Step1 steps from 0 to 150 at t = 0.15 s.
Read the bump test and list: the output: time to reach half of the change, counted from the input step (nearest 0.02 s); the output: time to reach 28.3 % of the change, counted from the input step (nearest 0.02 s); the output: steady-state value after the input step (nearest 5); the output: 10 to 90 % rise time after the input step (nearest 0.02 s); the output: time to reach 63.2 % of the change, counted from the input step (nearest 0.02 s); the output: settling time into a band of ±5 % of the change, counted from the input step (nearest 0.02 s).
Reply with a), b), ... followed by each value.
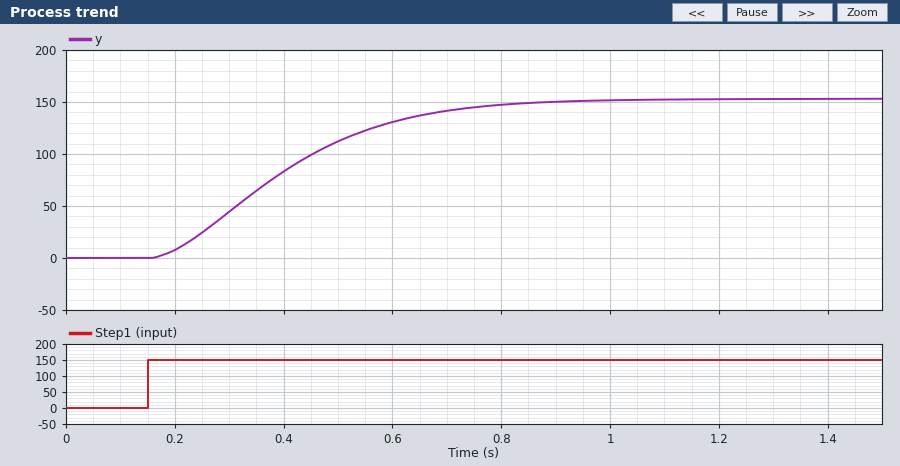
a) 0.24 s
b) 0.14 s
c) 155
d) 0.44 s
e) 0.30 s
f) 0.62 s
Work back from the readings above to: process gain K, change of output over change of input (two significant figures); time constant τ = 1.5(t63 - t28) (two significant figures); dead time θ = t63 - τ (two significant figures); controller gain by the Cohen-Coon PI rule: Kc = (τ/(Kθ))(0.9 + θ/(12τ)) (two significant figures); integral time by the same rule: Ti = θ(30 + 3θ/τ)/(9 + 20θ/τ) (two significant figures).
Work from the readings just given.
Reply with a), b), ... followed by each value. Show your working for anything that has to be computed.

a) (155 - 0) / 150 = 1.0
b) 1.5 × (0.3 - 0.14) = 0.24 s
c) 0.3 - 0.24 = 0.060 s
d) 0.24 / (1 × 0.06) × (0.9 + 0.06 / (12 × 0.24)) = 3.7
e) 0.06 × (30 + 3 × 0.06 / 0.24) / (9 + 20 × 0.06 / 0.24) = 0.13 s
